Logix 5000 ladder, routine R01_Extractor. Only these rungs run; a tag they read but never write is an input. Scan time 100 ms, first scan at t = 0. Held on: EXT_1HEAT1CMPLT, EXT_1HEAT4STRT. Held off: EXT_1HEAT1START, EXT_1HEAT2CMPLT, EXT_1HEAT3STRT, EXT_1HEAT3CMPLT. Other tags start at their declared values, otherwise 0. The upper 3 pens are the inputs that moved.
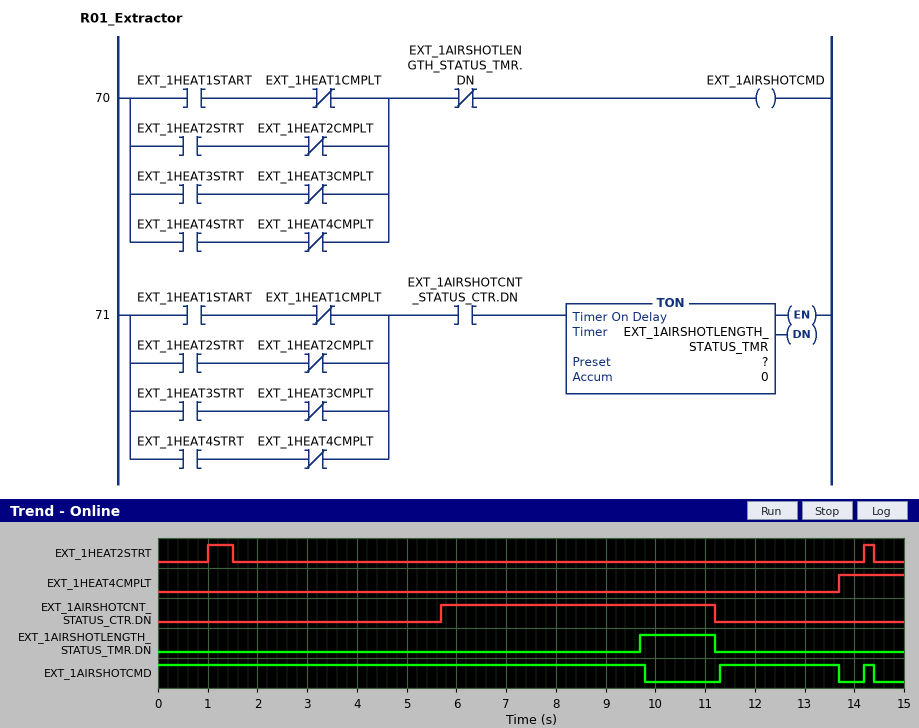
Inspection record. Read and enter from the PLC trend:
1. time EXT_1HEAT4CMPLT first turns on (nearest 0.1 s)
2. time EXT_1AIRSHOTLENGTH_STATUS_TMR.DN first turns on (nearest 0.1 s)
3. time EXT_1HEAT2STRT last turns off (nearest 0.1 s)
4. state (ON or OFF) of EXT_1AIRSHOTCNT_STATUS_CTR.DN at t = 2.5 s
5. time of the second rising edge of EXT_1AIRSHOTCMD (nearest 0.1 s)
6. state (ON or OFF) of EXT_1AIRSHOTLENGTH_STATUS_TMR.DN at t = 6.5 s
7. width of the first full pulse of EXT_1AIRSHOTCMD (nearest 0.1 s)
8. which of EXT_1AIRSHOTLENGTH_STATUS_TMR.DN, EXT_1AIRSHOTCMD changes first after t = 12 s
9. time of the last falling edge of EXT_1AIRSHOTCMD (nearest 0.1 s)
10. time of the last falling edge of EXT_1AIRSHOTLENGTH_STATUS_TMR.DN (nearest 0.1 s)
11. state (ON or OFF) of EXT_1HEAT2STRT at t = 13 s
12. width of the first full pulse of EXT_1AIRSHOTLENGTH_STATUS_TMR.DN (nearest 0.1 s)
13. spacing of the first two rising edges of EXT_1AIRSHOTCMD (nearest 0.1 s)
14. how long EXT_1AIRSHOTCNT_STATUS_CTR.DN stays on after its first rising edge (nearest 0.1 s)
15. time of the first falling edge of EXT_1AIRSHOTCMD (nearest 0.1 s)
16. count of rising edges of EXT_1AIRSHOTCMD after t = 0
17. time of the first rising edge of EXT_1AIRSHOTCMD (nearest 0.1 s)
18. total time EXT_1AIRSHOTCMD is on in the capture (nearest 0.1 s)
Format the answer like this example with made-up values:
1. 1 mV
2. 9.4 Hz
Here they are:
1. 13.7 s
2. 9.7 s
3. 14.4 s
4. OFF
5. 14.2 s
6. OFF
7. 2.4 s
8. EXT_1AIRSHOTCMD
9. 14.4 s
10. 11.2 s
11. OFF
12. 1.5 s
13. 2.9 s
14. 5.5 s
15. 9.8 s
16. 2
17. 11.3 s
18. 12.4 s
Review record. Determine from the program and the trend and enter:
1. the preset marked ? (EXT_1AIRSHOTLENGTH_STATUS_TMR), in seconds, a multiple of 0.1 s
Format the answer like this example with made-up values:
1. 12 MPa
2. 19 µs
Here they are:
1. 4.0 s
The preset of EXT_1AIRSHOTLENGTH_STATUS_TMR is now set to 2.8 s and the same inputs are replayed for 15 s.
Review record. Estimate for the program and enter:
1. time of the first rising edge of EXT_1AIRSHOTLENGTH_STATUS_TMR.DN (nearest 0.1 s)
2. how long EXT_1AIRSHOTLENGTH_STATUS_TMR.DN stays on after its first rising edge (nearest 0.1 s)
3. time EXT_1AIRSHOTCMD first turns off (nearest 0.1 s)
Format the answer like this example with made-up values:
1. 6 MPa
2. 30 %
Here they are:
1. 8.5 s
2. 2.7 s
3. 8.6 s
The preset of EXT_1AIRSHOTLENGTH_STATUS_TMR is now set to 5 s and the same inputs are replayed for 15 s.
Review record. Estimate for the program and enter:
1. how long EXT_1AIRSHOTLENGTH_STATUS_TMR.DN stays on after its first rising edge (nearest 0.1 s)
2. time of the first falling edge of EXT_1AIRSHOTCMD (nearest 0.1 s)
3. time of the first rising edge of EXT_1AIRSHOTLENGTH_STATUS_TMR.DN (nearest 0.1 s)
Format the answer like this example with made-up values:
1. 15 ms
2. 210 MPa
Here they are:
1. 0.5 s
2. 10.8 s
3. 10.7 s
